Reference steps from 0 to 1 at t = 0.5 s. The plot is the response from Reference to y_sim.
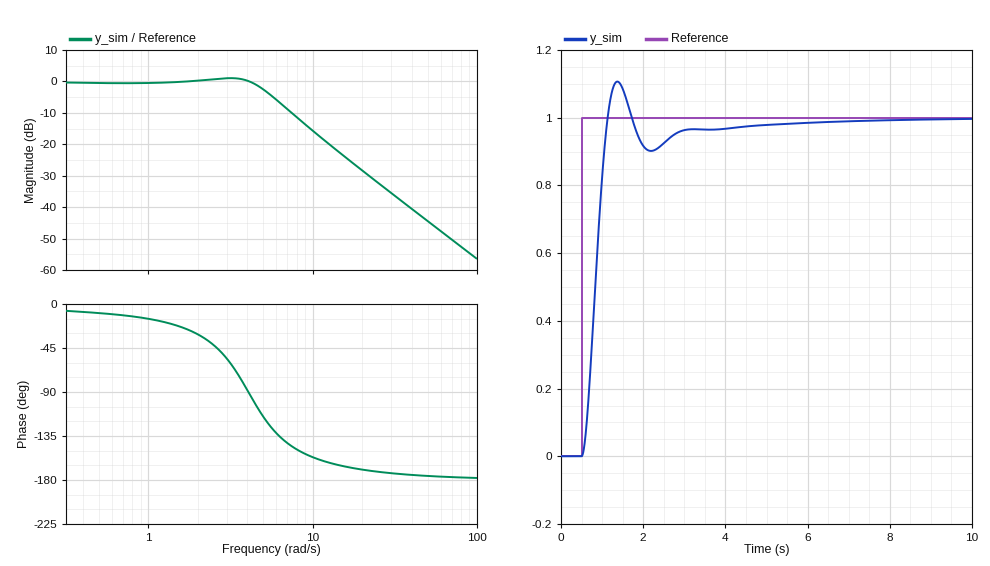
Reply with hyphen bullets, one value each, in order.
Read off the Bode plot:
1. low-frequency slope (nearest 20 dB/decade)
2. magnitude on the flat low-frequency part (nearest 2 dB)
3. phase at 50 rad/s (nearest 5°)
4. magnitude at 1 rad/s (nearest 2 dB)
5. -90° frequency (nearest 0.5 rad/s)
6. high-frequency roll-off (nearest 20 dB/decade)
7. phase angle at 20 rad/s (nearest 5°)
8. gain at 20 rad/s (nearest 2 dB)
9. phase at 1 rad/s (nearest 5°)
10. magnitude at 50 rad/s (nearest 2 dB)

- 0 dB/decade
- 0 dB
- -175°
- 0 dB
- 4.0 rad/s
- -40 dB/decade
- -170°
- -28 dB
- -15°
- -44 dB
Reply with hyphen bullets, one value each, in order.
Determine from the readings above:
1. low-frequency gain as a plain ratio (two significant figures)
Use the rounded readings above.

- 1.0
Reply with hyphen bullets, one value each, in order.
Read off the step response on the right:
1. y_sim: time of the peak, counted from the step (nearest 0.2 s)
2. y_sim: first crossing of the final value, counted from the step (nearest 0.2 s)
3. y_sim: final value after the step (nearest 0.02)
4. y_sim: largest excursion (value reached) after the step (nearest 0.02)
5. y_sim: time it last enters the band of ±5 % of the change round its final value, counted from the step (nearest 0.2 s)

- 0.8 s
- 0.6 s
- 1.00
- 1.10
- 2.2 s
